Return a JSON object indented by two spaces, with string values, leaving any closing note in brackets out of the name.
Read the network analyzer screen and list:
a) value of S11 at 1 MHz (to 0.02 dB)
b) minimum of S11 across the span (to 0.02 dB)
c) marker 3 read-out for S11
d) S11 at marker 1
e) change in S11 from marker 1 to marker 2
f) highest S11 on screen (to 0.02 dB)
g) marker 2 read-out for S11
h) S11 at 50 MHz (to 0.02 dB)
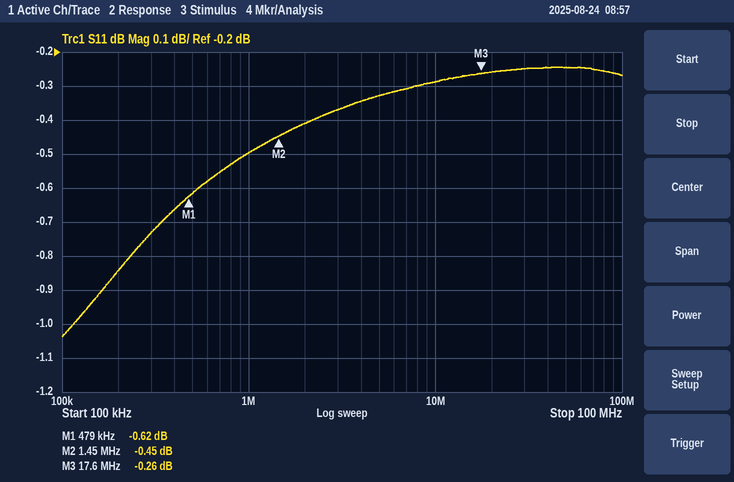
{
  "value of S11 at 1 MHz": "-0.50 dB",
  "minimum of S11 across the span": "-1.04 dB",
  "marker 3 read-out for S11": "-0.26 dB",
  "S11 at marker 1": "-0.62 dB",
  "change in S11 from marker 1 to marker 2": "0.17 dB",
  "highest S11 on screen": "-0.24 dB",
  "marker 2 read-out for S11": "-0.45 dB",
  "S11 at 50 MHz": "-0.24 dB"
}
